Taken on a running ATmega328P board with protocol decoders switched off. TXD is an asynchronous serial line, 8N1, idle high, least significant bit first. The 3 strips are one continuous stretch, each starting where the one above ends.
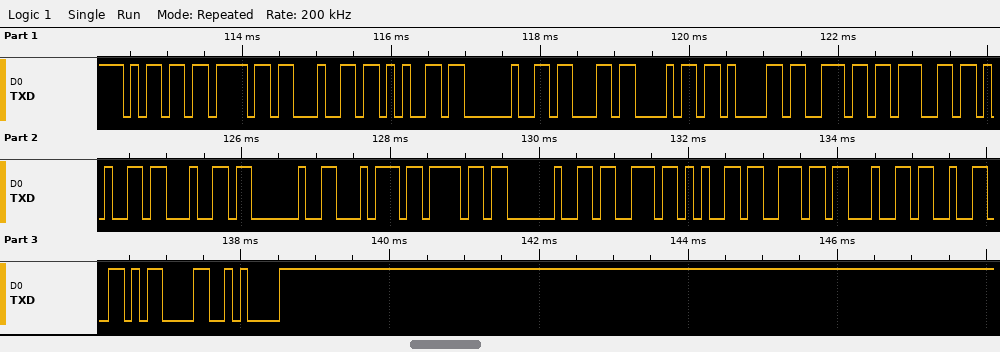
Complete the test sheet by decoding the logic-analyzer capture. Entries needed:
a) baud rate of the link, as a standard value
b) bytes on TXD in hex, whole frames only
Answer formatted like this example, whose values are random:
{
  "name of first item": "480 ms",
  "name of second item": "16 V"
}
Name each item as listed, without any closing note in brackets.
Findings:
{
  "baud rate of the link, as a standard value": "9600 baud",
  "bytes on TXD in hex, whole frames only": "6D 6F 64 65 20 63 68 61 6E 67 65 64 20 74 6F 20 73 65 6E 64 32 0D 0A"
}
